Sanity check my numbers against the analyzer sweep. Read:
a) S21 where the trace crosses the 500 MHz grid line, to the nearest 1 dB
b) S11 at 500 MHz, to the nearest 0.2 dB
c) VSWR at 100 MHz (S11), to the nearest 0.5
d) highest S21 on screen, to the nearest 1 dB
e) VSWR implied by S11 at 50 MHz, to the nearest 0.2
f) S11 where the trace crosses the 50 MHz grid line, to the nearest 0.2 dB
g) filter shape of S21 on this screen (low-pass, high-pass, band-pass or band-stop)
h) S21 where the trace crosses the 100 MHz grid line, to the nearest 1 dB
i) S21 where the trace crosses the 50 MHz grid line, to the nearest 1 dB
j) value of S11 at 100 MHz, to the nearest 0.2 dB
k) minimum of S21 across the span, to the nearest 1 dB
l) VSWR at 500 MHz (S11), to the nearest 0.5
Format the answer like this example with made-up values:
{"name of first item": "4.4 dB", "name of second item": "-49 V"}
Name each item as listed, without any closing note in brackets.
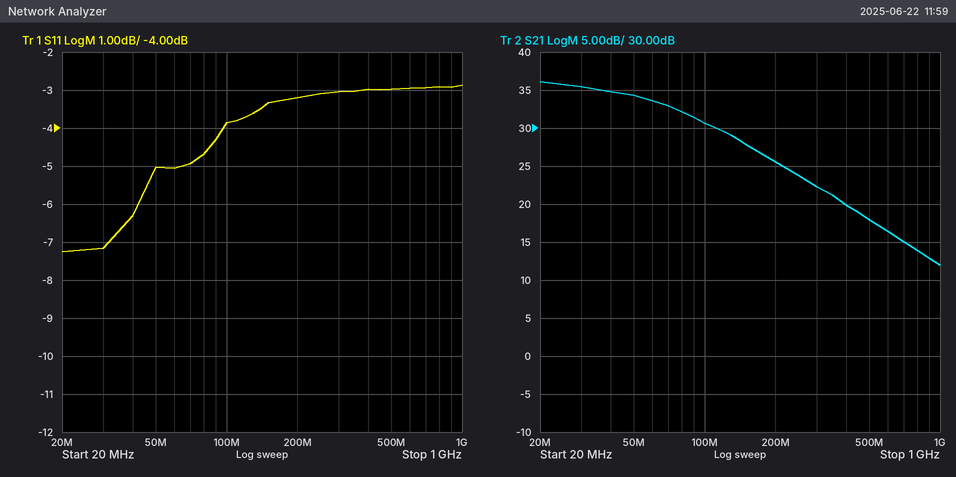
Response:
{"S21 where the trace crosses the 500 MHz grid line, to the nearest 1 dB": "18 dB", "S11 at 500 MHz, to the nearest 0.2 dB": "-3.0 dB", "VSWR at 100 MHz (S11), to the nearest 0.5": "4.5", "highest S21 on screen, to the nearest 1 dB": "36 dB", "VSWR implied by S11 at 50 MHz, to the nearest 0.2": "3.6", "S11 where the trace crosses the 50 MHz grid line, to the nearest 0.2 dB": "-5.0 dB", "filter shape of S21 on this screen": "low-pass", "S21 where the trace crosses the 100 MHz grid line, to the nearest 1 dB": "31 dB", "S21 where the trace crosses the 50 MHz grid line, to the nearest 1 dB": "34 dB", "value of S11 at 100 MHz, to the nearest 0.2 dB": "-3.8 dB", "minimum of S21 across the span, to the nearest 1 dB": "12 dB", "VSWR at 500 MHz (S11), to the nearest 0.5": "6.0"}
